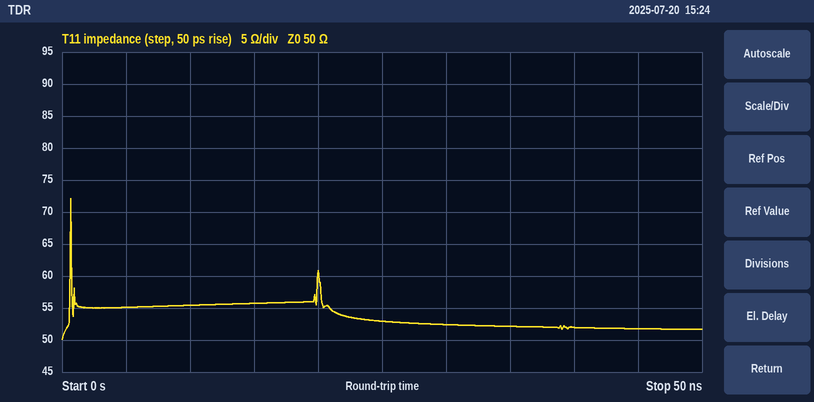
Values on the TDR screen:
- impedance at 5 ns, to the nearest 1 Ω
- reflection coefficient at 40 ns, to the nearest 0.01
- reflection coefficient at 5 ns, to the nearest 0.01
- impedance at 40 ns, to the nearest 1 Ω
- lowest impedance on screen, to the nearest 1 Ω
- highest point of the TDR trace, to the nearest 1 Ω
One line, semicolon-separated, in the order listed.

55 Ω; +0.02; +0.05; 52 Ω; 50 Ω; 72 Ω
